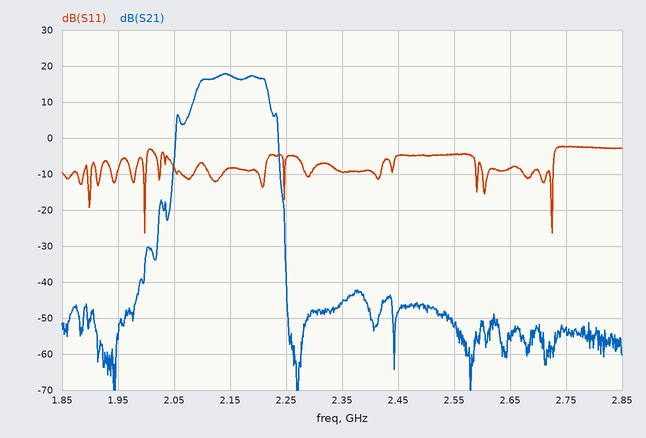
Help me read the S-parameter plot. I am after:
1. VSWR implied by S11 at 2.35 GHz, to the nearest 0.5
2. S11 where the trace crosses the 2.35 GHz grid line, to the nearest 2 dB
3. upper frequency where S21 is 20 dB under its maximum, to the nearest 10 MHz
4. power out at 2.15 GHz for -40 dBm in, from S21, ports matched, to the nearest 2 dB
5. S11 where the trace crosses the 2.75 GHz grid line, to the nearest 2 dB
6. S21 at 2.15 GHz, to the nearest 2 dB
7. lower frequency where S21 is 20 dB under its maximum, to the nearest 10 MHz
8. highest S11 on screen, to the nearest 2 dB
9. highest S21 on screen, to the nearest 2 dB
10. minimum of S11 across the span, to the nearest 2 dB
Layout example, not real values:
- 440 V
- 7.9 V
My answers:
- 2.0
- -10 dB
- 2.24 GHz
- -22 dBm
- -2 dB
- 18 dB
- 2.05 GHz
- -2 dB
- 18 dB
- -26 dB
